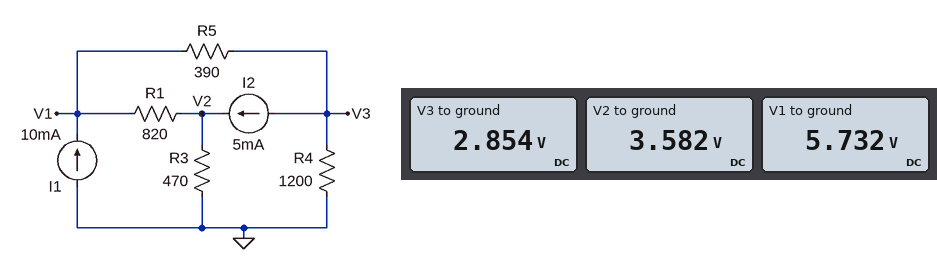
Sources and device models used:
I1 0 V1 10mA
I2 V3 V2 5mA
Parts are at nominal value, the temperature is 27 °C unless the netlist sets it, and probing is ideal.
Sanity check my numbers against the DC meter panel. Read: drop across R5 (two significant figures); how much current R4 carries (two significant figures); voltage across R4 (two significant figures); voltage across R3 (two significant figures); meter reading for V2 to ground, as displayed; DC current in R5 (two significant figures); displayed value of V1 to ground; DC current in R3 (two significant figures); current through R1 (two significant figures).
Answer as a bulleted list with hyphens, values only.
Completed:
- 2.9 V
- 2.4 mA
- 2.9 V
- 3.6 V
- 3.582 V
- 7.4 mA
- 5.732 V
- 7.6 mA
- 2.6 mA
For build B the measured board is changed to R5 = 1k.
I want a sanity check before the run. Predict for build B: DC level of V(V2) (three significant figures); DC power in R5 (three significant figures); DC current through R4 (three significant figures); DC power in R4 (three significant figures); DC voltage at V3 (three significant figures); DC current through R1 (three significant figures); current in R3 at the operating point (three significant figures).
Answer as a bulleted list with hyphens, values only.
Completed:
- 4.19 V
- 37.1 mW
- 1.09 mA
- 1.42 mW
- 1.31 V
- 3.91 mA
- 8.91 mA
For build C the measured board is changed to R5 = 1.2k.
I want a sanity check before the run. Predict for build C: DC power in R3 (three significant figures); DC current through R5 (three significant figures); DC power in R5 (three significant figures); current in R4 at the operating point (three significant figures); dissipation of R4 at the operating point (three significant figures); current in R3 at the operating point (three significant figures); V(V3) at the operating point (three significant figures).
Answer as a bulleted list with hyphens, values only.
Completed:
- 40.1 mW
- 5.76 mA
- 39.8 mW
- 759 µA
- 691 µW
- 9.24 mA
- 911 mV
